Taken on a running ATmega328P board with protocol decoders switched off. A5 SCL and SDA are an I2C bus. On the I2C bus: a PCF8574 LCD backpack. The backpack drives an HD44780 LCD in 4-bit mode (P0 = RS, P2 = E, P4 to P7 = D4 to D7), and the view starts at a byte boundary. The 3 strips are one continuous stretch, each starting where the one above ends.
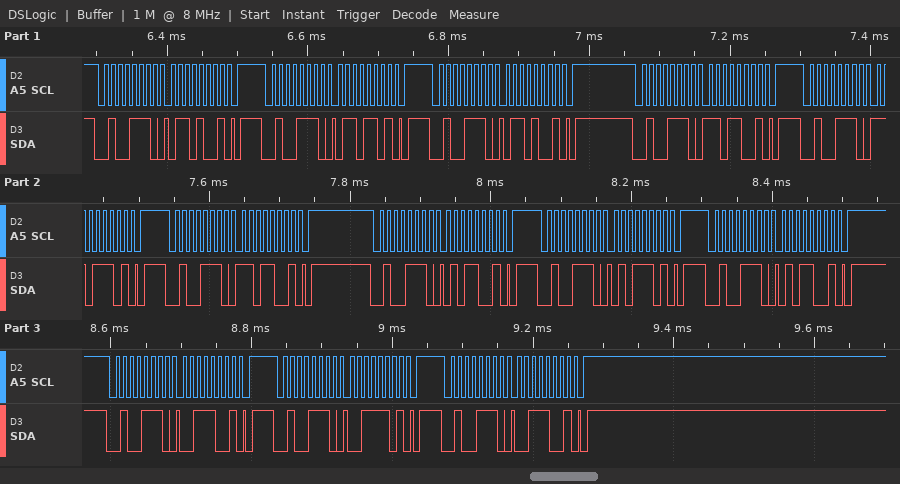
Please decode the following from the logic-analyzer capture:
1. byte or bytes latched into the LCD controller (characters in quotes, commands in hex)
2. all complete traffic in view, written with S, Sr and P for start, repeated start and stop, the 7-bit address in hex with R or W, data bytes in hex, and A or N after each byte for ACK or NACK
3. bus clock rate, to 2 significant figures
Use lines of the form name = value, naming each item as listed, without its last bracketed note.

byte or bytes latched into the LCD controller = 'm' 'S'
all complete traffic in view, written with S, Sr and P for start, repeated start and stop, the 7-bit address in hex with R or W, data bytes in hex, and A or N after each byte for ACK or NACK = S 27W A 69 A P S 27W A 6D A P S 27W A 69 A P S 27W A D9 A P S 27W A DD A P S 27W A D9 A P S 27W A 59 A P S 27W A 5D A P S 27W A 59 A P S 27W A 39 A P S 27W A 3D A P S 27W A 39 A P
bus clock rate, to 2 significant figures = 100 kHz
